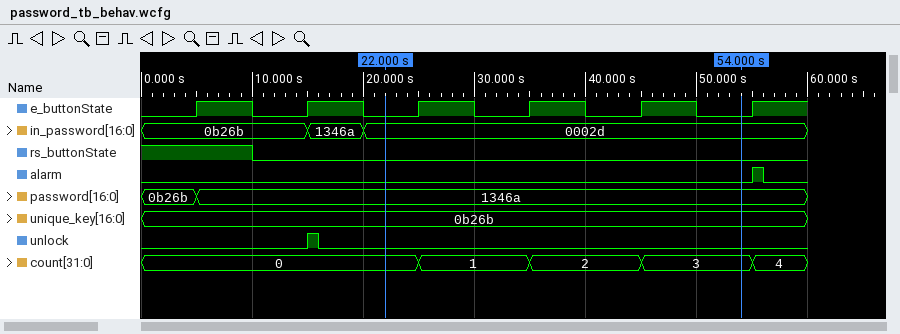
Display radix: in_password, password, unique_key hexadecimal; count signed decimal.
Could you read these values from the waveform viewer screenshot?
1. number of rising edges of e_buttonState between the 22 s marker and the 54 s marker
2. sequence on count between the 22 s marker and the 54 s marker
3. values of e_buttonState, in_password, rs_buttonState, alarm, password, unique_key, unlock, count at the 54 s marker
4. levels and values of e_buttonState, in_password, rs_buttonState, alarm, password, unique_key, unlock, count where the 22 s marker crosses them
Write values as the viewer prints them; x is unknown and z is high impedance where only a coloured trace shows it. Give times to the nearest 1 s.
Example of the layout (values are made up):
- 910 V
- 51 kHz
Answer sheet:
- 3
- 0, 1, 2, 3
- e_buttonState=0, in_password=0002d, rs_buttonState=0, alarm=0, password=1346a, unique_key=0b26b, unlock=0, count=3
- e_buttonState=0, in_password=0002d, rs_buttonState=0, alarm=0, password=1346a, unique_key=0b26b, unlock=0, count=0
